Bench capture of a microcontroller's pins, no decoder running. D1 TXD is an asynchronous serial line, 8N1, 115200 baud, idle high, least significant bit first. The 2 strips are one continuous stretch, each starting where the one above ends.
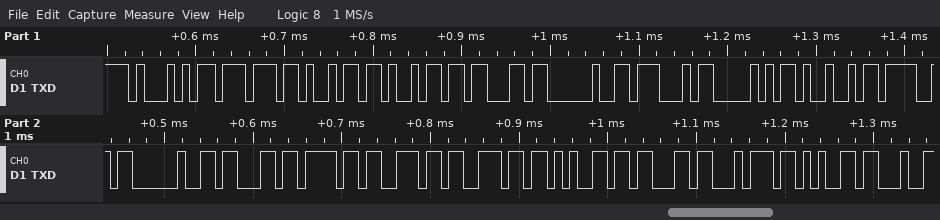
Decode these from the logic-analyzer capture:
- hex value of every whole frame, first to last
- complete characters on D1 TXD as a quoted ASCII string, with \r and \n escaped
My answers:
51 77 69 69 63 20 47 50 49 4F 20 63 6F 6E 6E 65 63 74 65
"Qwiic GPIO connecte"
